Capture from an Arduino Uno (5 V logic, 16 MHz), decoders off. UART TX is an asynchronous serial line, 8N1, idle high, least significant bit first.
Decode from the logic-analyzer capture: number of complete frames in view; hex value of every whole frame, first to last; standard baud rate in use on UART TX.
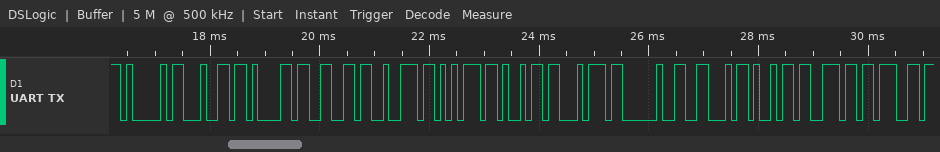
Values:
13
0x41 0x64 0x61 0x66 0x72 0x75 0x69 0x74 0x20 0x46 0x69 0x6E 0x67
9600 baud
